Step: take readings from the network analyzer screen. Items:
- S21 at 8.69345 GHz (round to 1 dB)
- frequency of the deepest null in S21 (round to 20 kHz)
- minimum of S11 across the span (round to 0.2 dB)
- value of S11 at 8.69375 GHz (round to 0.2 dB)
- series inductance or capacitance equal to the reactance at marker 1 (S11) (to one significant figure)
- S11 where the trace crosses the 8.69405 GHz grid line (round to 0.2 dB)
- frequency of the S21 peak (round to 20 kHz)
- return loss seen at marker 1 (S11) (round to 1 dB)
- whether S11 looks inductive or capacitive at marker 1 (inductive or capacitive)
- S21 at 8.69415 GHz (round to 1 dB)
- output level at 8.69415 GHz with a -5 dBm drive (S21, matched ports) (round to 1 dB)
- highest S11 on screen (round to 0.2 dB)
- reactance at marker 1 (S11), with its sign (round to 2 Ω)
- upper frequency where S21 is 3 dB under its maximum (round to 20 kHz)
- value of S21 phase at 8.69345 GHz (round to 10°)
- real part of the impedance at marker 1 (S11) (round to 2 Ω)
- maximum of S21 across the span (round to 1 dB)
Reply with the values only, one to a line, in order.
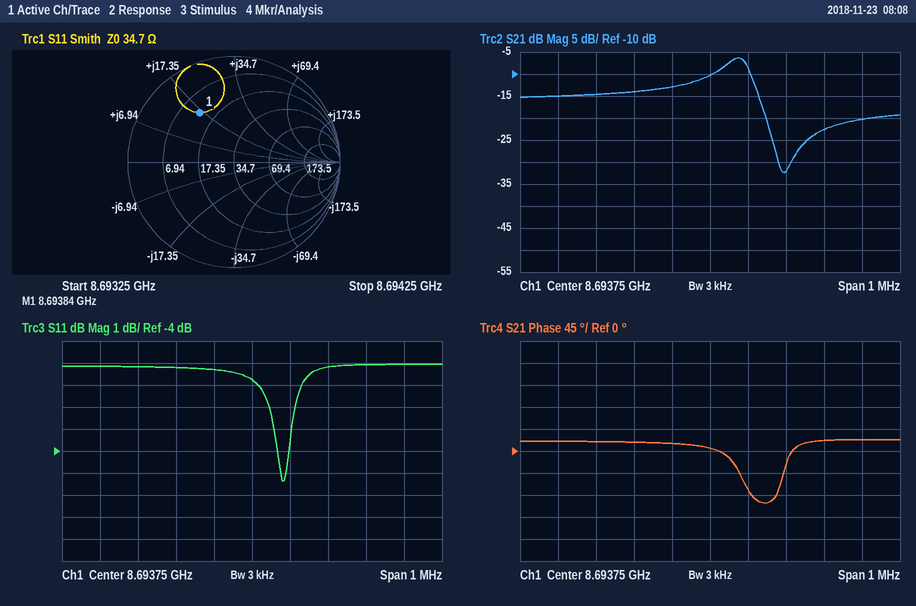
-15 dB
8.69394 GHz
-5.4 dB
-0.8 dB
300 pH
0.0 dB
8.69382 GHz
5 dB
inductive
-20 dB
-25 dBm
0.0 dB
+16 Ω
8.69386 GHz
20°
12 Ω
-6 dB
